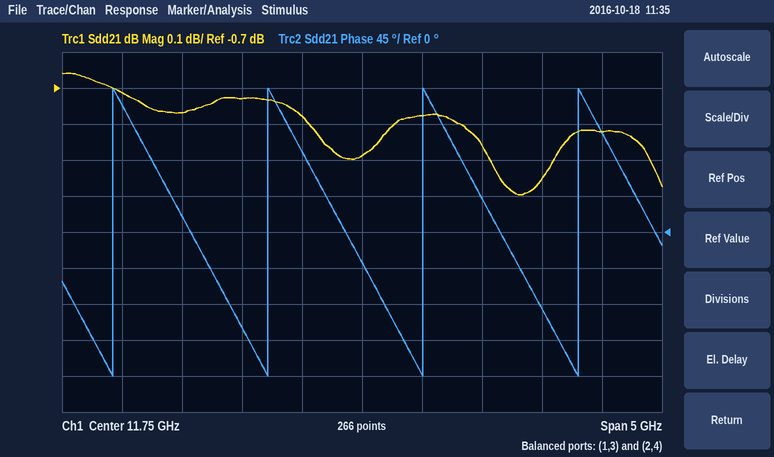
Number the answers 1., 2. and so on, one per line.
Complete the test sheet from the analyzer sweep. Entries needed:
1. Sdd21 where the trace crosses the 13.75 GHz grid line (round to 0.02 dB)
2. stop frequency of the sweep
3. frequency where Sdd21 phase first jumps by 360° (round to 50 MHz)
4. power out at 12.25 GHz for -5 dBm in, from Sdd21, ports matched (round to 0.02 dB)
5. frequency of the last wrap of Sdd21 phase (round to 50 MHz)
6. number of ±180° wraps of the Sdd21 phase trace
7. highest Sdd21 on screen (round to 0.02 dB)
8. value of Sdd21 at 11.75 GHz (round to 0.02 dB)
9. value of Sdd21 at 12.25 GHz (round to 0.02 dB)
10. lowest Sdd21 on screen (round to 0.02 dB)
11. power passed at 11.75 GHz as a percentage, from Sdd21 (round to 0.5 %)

1. -0.82 dB
2. 14.25 GHz
3. 9.65 GHz
4. -5.78 dBm
5. 13.55 GHz
6. 4
7. -0.66 dB
8. -0.88 dB
9. -0.78 dB
10. -1.00 dB
11. 81.5 %
